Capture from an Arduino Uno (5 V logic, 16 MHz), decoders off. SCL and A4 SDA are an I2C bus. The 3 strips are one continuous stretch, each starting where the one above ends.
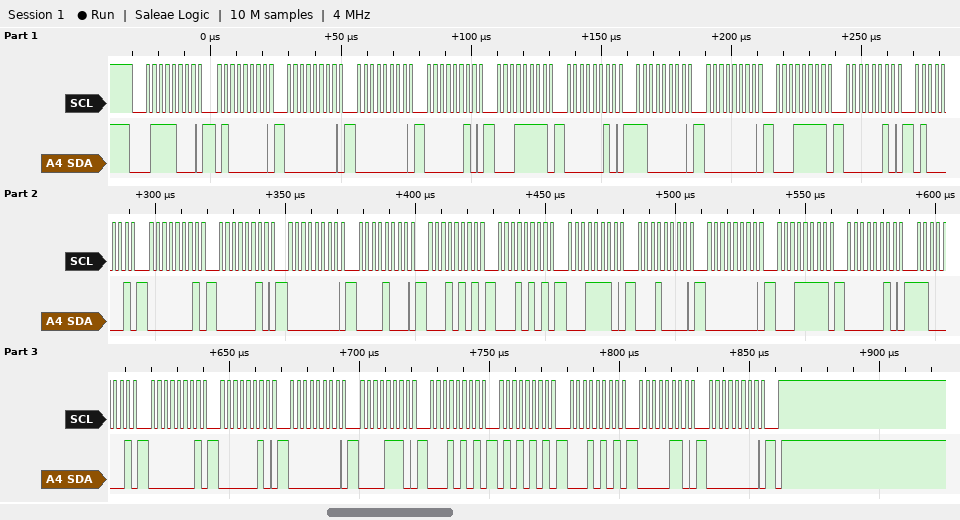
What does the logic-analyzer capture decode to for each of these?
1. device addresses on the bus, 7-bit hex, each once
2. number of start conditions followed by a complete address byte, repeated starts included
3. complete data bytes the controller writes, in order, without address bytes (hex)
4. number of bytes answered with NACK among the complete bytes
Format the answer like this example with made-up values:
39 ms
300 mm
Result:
0x3C
1
40 00 00 02 1F 02 C0 00 1F 02 41 01 02 00 08 15 15 1E 10 00 1F 02 C1 01 02 00 0E 15 55 15 06 00
0
